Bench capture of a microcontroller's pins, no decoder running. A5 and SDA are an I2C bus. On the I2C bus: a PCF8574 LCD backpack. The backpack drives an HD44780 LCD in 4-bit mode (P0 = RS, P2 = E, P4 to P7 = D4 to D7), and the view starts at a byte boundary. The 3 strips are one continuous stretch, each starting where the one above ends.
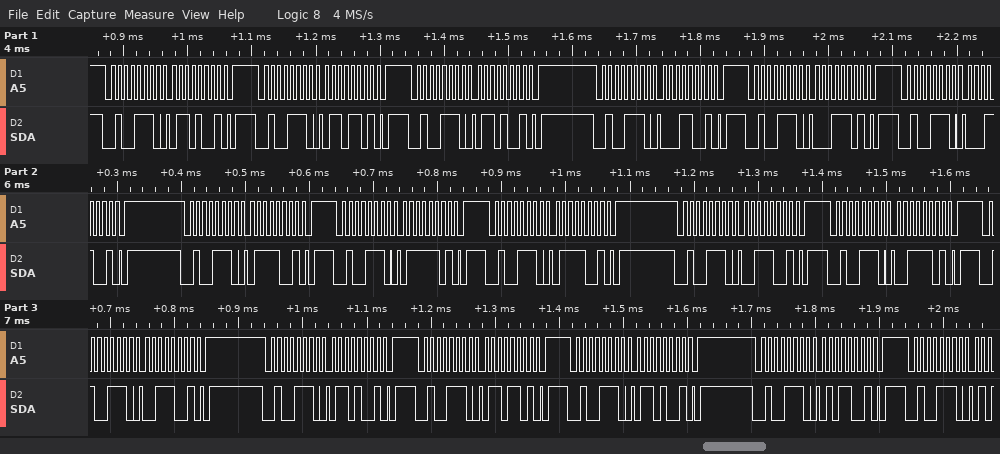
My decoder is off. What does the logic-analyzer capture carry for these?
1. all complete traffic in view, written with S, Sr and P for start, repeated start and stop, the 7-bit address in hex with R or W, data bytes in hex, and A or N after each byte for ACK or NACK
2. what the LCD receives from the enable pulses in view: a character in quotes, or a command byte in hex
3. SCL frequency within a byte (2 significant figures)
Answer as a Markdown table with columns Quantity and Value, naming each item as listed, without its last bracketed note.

| Quantity | Value |
|---|---|
| all complete traffic in view, written with S, Sr and P for start, repeated start and stop, the 7-bit address in hex with R or W, data bytes in hex, and A or N after each byte for ACK or NACK | S 27W A 69 A P S 27W A 6D A P S 27W A 69 A P S 27W A 19 A P S 27W A 1D A P S 27W A 19 A P S 27W A 79 A P S 27W A 7D A P S 27W A 79 A P S 27W A 39 A P S 27W A 3D A P S 27W A 39 A P S 27W A 69 A P S 27W A 6D A P S 27W A 69 A P S 27W A 59 A P S 27W A |
| what the LCD receives from the enable pulses in view: a character in quotes, or a command byte in hex | 'a' 's' |
| SCL frequency within a byte | 100 kHz |
